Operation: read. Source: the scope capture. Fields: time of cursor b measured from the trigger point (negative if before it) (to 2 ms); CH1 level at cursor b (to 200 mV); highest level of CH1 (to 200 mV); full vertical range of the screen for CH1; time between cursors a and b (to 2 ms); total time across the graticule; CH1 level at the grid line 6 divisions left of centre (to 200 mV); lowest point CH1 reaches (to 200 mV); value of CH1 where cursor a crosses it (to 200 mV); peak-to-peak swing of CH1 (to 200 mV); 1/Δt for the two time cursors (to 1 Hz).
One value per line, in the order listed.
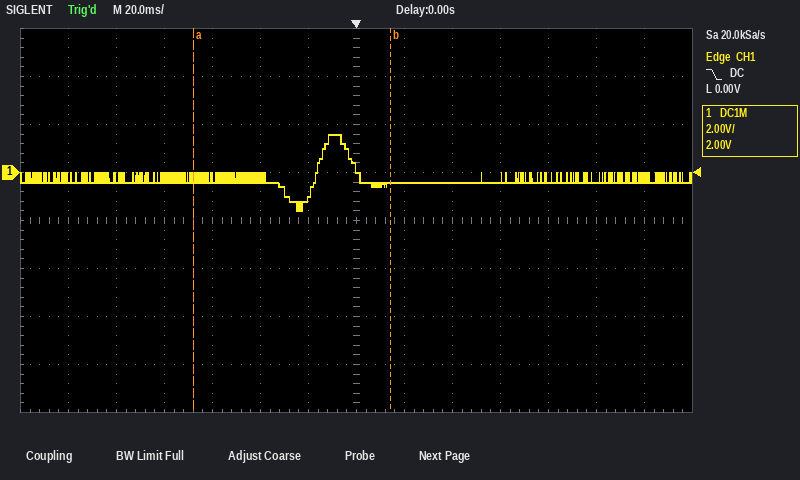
+14 ms
-400 mV
1.6 V
16 V
82 ms
280 ms
-200 mV
-1.6 V
-200 mV
3.2 V
12 Hz
